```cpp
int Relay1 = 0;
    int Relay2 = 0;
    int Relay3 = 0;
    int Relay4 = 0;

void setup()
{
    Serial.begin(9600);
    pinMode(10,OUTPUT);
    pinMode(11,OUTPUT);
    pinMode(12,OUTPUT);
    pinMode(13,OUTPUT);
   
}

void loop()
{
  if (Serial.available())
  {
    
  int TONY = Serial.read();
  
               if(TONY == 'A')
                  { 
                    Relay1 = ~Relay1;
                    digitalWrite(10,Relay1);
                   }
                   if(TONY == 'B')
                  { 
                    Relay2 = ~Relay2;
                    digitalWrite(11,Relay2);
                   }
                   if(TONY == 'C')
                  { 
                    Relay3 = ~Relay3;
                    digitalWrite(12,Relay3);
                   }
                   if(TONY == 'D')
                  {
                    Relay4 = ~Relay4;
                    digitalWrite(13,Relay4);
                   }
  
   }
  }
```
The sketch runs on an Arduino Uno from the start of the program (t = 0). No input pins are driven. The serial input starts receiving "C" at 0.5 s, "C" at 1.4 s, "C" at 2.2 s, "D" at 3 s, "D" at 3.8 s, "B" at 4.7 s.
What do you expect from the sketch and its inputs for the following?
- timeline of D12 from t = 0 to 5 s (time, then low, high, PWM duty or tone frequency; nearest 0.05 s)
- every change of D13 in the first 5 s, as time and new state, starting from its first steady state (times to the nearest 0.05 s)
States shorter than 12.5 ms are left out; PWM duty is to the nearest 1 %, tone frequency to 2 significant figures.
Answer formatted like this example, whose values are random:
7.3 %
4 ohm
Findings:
0 s low; 0.5 s high; 1.4 s low; 2.2 s high
0 s low; 3 s high; 3.8 s low
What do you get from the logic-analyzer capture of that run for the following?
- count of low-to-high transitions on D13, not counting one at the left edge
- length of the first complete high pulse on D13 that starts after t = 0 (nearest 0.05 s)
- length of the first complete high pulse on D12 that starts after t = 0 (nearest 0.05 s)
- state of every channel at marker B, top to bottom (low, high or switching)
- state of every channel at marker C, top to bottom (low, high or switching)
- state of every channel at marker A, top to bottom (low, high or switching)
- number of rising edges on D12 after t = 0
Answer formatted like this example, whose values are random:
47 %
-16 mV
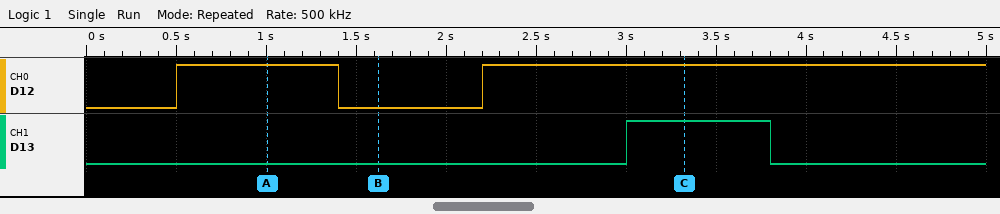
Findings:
1
0.80 s
0.90 s
D12 low, D13 low
D12 high, D13 high
D12 high, D13 low
2
